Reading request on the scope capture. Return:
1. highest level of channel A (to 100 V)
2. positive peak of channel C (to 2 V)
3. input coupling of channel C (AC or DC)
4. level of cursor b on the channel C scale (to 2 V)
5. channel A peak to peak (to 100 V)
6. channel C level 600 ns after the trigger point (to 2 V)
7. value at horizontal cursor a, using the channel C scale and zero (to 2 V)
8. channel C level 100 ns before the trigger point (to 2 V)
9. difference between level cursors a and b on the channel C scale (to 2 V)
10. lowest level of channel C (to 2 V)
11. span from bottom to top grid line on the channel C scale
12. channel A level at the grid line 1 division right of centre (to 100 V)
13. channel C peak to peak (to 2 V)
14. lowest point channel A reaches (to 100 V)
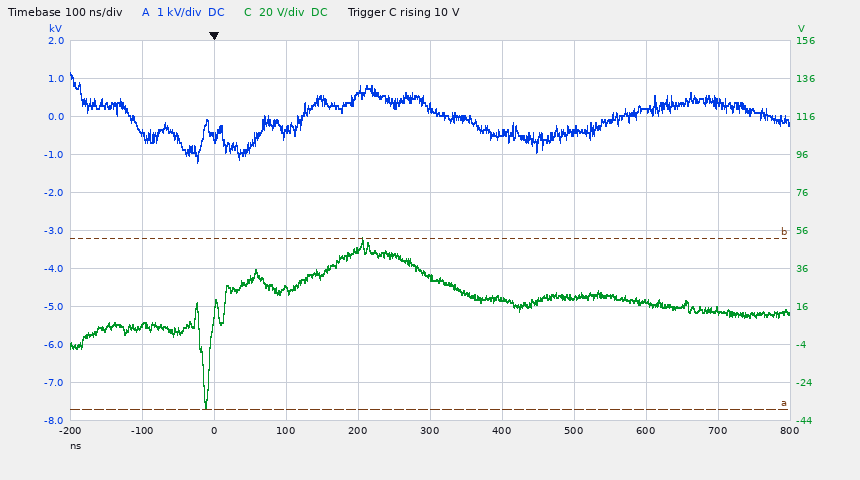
1.2 kV
52 V
DC
52 V
2.4 kV
18 V
-38 V
6 V
90 V
-38 V
200 V
-400 V
90 V
-1.2 kV
